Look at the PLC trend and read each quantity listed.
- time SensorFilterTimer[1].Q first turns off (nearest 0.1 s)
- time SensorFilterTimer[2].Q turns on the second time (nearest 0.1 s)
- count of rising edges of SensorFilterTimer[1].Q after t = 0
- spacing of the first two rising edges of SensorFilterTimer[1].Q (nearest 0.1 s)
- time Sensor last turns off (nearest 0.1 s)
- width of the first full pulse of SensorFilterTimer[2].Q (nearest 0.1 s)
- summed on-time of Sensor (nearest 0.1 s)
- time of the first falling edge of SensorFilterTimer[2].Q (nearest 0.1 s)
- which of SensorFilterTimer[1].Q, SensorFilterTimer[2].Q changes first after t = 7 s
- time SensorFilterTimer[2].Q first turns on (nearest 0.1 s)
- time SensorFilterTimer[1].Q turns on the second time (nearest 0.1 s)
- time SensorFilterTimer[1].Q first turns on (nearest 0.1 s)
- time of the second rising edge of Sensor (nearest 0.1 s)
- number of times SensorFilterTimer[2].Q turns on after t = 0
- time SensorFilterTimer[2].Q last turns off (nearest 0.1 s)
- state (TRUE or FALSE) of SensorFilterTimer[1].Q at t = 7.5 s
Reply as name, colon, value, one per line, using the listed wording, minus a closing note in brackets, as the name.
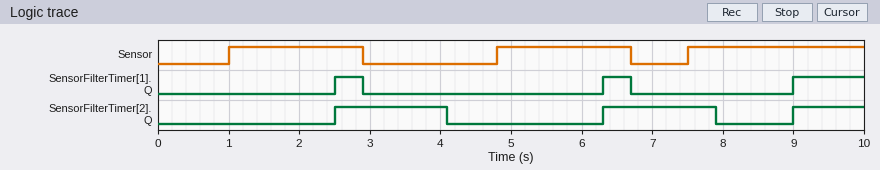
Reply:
time SensorFilterTimer[1].Q first turns off: 2.9 s
time SensorFilterTimer[2].Q turns on the second time: 6.3 s
count of rising edges of SensorFilterTimer[1].Q after t = 0: 3
spacing of the first two rising edges of SensorFilterTimer[1].Q: 3.8 s
time Sensor last turns off: 6.7 s
width of the first full pulse of SensorFilterTimer[2].Q: 1.6 s
summed on-time of Sensor: 6.3 s
time of the first falling edge of SensorFilterTimer[2].Q: 4.1 s
which of SensorFilterTimer[1].Q, SensorFilterTimer[2].Q changes first after t = 7 s: SensorFilterTimer[2].Q
time SensorFilterTimer[2].Q first turns on: 2.5 s
time SensorFilterTimer[1].Q turns on the second time: 6.3 s
time SensorFilterTimer[1].Q first turns on: 2.5 s
time of the second rising edge of Sensor: 4.8 s
number of times SensorFilterTimer[2].Q turns on after t = 0: 3
time SensorFilterTimer[2].Q last turns off: 7.9 s
state (TRUE or FALSE) of SensorFilterTimer[1].Q at t = 7.5 s: FALSE
